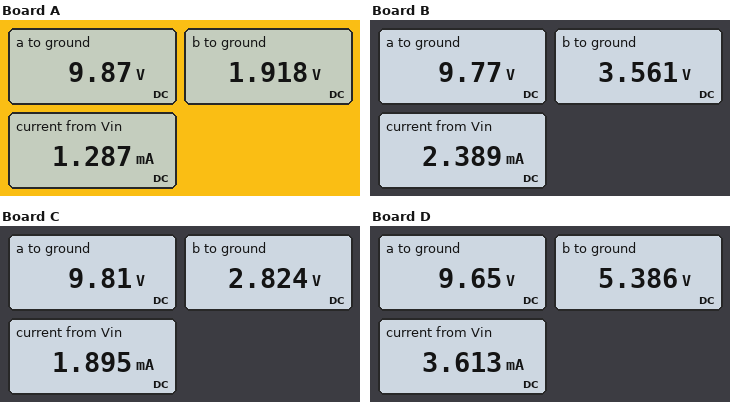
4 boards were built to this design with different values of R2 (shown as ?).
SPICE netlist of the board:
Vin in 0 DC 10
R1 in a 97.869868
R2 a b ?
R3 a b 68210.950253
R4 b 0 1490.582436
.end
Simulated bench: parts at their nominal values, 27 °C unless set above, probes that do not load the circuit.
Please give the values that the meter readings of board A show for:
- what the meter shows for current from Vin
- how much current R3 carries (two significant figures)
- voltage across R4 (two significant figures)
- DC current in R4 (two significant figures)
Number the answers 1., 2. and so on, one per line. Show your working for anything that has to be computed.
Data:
1. 1.287 mA
2. (9.87 V - 1.918 V) / 68.21 kΩ = 120 µA
3. 1.918 V = 1.9 V
4. (1.918 V) / 1.491 kΩ = 1.3 mA
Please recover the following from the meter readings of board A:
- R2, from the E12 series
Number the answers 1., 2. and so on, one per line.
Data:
1. 6.8 kΩ
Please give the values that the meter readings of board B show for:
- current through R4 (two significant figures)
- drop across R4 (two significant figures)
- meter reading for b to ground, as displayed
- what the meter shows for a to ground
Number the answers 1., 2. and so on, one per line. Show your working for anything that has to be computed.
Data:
1. (3.561 V) / 1.491 kΩ = 2.4 mA
2. 3.561 V = 3.6 V
3. 3.561 V
4. 9.77 V
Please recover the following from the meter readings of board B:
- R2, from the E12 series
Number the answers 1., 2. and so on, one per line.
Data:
1. 2.7 kΩ
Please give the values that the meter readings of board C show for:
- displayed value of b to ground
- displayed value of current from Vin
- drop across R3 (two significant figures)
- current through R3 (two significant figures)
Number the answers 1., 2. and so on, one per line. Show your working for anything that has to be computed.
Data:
1. 2.824 V
2. 1.895 mA
3. 9.81 V - 2.824 V = 7.0 V
4. (9.81 V - 2.824 V) / 68.21 kΩ = 100 µA
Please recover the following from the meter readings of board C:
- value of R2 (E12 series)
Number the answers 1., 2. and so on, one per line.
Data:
1. 3.9 kΩ
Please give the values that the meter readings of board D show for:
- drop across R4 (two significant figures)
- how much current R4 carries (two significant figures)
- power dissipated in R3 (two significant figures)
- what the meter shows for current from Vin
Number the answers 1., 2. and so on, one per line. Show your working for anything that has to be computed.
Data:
1. 5.386 V = 5.4 V
2. (5.386 V) / 1.491 kΩ = 3.6 mA
3. (9.65 V - 5.386 V)^2 / 68.21 kΩ = 270 µW
4. 3.613 mA
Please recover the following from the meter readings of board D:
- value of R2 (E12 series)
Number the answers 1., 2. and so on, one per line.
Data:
1. 1.2 kΩ
